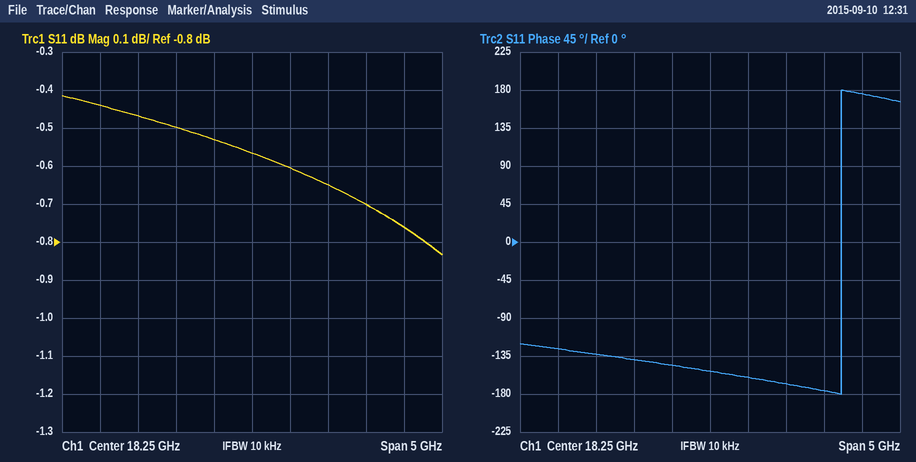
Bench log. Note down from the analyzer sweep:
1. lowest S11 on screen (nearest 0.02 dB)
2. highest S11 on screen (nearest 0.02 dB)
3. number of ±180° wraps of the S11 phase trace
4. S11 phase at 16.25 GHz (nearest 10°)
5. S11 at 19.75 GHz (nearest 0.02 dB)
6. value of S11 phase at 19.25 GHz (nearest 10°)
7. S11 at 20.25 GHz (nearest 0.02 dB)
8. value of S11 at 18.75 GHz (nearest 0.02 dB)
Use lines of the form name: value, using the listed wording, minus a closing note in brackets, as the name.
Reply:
lowest S11 on screen: -0.84 dB
highest S11 on screen: -0.42 dB
number of ±180° wraps of the S11 phase trace: 1
S11 phase at 16.25 GHz: -130°
S11 at 19.75 GHz: -0.70 dB
value of S11 phase at 19.25 GHz: -170°
S11 at 20.25 GHz: -0.76 dB
value of S11 at 18.75 GHz: -0.60 dB
